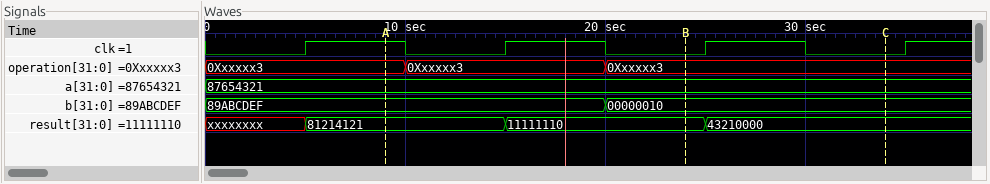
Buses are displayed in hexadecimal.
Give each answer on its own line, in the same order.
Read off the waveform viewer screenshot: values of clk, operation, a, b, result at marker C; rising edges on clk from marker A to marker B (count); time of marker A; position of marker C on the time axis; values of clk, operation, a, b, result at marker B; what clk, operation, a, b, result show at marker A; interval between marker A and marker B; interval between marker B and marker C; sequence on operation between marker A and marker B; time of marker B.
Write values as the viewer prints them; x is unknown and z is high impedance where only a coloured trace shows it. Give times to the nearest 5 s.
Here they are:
clk=0, operation=0Xxxxxx3, a=87654321, b=00000010, result=43210000
1
10 s
35 s
clk=0, operation=0Xxxxxx3, a=87654321, b=00000010, result=11111110
clk=1, operation=0Xxxxxx3, a=87654321, b=89ABCDEF, result=81214121
15 s
10 s
0Xxxxxx3, 0Xxxxxx3, 0Xxxxxx3
25 s
